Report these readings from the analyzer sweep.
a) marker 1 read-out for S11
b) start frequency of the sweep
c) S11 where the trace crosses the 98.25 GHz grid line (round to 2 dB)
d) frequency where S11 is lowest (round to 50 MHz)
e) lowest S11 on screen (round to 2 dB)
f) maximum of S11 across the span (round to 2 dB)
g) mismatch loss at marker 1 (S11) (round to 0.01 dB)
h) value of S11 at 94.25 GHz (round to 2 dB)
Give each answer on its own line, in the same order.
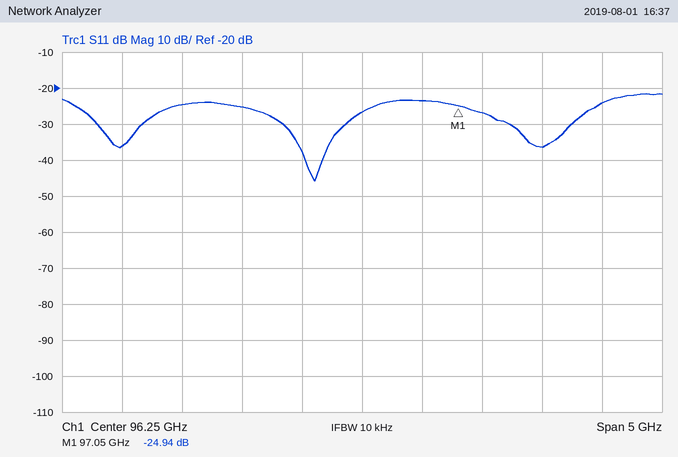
-24.94 dB
93.75 GHz
-24 dB
95.85 GHz
-46 dB
-22 dB
0.01 dB
-36 dB
